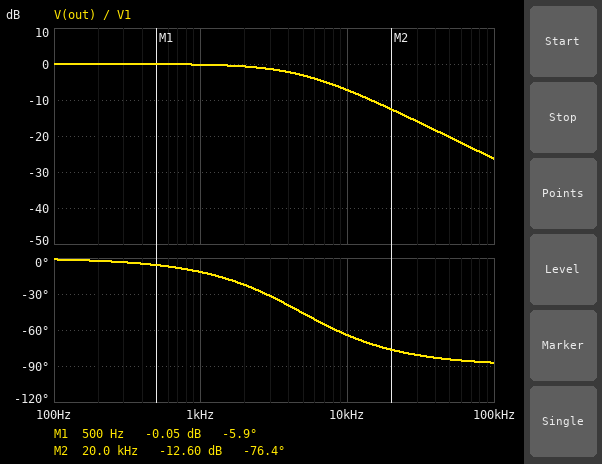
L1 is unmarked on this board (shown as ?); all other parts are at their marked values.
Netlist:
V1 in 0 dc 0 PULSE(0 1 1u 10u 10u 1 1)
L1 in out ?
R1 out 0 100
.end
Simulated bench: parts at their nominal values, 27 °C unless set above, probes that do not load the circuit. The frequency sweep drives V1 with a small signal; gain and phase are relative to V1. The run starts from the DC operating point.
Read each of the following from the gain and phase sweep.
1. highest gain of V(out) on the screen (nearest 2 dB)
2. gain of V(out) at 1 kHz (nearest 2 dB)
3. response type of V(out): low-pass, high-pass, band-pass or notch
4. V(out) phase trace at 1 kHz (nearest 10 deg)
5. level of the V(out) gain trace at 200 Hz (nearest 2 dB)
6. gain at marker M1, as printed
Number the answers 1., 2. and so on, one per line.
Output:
1. 0 dB
2. 0 dB
3. low-pass
4. -10 deg
5. 0 dB
6. -0.05 dB
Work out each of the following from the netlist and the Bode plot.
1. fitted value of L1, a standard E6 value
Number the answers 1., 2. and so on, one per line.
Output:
1. 3.3 mH
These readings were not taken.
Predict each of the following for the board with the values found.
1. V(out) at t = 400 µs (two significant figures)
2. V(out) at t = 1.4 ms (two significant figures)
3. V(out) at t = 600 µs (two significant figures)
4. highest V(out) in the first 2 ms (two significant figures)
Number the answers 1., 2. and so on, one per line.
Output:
1. 1.0 V
2. 1.0 V
3. 1.0 V
4. 1.0 V
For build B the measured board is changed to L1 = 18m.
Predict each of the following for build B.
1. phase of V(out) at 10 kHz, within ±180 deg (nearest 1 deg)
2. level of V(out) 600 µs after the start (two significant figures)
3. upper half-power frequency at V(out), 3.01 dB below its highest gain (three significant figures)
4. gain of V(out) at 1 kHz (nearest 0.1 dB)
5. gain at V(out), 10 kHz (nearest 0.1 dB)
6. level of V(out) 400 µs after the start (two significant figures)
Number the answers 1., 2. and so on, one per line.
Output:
1. -85 deg
2. 960 mV
3. 884 Hz
4. -3.6 dB
5. -21.1 dB
6. 890 mV
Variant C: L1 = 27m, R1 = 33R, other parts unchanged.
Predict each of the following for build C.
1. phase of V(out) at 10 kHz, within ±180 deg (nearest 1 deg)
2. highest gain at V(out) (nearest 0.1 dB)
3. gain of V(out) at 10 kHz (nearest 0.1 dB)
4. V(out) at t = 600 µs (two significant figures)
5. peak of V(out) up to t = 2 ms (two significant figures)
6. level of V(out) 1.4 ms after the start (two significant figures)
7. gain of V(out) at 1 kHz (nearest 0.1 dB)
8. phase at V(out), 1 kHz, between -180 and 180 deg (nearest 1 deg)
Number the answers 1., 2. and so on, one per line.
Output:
1. -89 deg
2. 0 dB
3. -34.2 dB
4. 520 mV
5. 910 mV
6. 820 mV
7. -14.4 dB
8. -79 deg
